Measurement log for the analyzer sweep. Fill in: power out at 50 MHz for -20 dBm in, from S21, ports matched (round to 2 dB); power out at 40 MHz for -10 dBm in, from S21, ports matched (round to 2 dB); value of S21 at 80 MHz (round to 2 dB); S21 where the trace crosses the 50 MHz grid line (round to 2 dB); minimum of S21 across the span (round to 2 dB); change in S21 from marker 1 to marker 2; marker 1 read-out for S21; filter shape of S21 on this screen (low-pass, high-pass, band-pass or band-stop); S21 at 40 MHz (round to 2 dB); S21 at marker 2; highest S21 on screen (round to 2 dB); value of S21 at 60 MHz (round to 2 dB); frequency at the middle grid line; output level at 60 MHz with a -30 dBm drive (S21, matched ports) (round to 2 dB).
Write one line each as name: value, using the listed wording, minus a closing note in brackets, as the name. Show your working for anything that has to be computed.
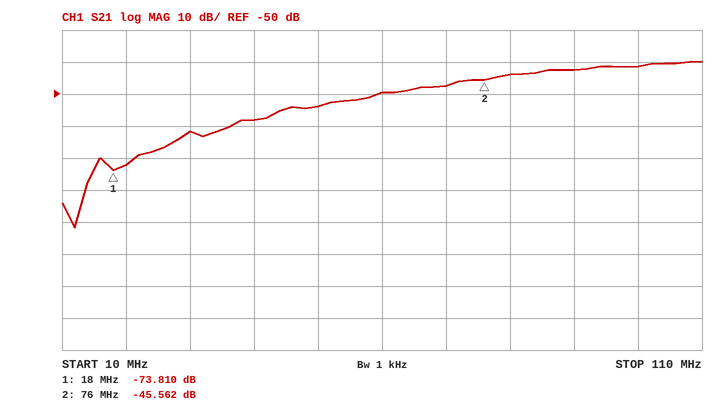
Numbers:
power out at 50 MHz for -20 dBm in, from S21, ports matched: -20 dBm + (-54 dB) = -74 dBm
power out at 40 MHz for -10 dBm in, from S21, ports matched: -10 dBm + (-58 dB) = -68 dBm
value of S21 at 80 MHz: -44 dB
S21 where the trace crosses the 50 MHz grid line: -54 dB
minimum of S21 across the span: -92 dB
change in S21 from marker 1 to marker 2: -45.562 − (-73.81) = 28.248 dB
marker 1 read-out for S21: -73.810 dB
filter shape of S21 on this screen: high-pass
S21 at 40 MHz: -58 dB
S21 at marker 2: -45.562 dB
highest S21 on screen: -40 dB
value of S21 at 60 MHz: -50 dB
frequency at the middle grid line: 60 MHz
output level at 60 MHz with a -30 dBm drive (S21, matched ports): -30 dBm + (-50 dB) = -80 dBm
